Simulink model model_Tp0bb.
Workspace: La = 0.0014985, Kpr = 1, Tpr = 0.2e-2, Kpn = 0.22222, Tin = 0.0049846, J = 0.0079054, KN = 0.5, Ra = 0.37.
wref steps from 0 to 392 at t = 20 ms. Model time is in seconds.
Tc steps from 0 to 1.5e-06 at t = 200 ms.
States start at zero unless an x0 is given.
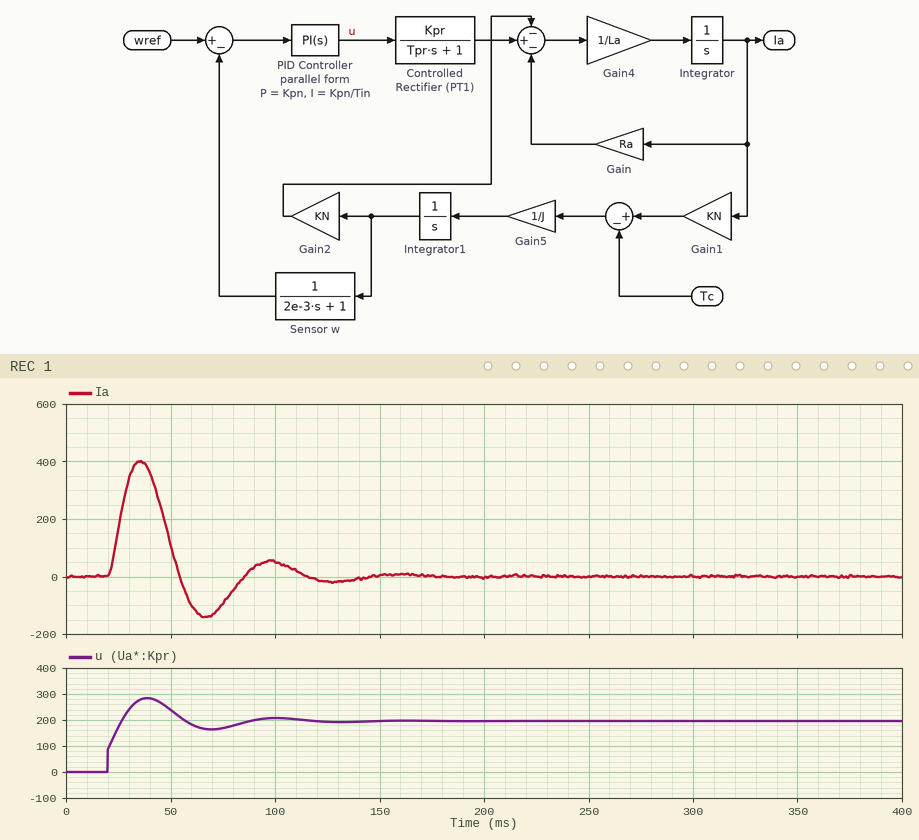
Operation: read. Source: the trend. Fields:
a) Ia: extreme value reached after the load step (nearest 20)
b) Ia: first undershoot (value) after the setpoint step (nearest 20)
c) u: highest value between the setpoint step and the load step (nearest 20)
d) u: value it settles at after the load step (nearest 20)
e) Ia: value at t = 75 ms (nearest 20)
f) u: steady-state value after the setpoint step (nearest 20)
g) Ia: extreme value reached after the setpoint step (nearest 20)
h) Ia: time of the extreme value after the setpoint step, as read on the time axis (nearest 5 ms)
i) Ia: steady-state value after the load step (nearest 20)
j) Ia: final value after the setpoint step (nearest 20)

0
-140
280
200
-100
200
400
35 ms
0
0
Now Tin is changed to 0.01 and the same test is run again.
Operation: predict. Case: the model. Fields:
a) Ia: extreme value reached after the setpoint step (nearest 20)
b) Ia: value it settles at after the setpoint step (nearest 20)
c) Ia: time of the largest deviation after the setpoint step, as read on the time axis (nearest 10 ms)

260
0
30 ms
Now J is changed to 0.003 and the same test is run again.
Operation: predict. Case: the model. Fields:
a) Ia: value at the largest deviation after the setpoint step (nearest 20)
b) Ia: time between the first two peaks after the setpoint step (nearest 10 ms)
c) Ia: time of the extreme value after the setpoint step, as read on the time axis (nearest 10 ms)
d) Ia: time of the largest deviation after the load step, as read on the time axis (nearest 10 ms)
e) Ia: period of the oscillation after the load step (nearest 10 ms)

240
30 ms
30 ms
220 ms
30 ms
